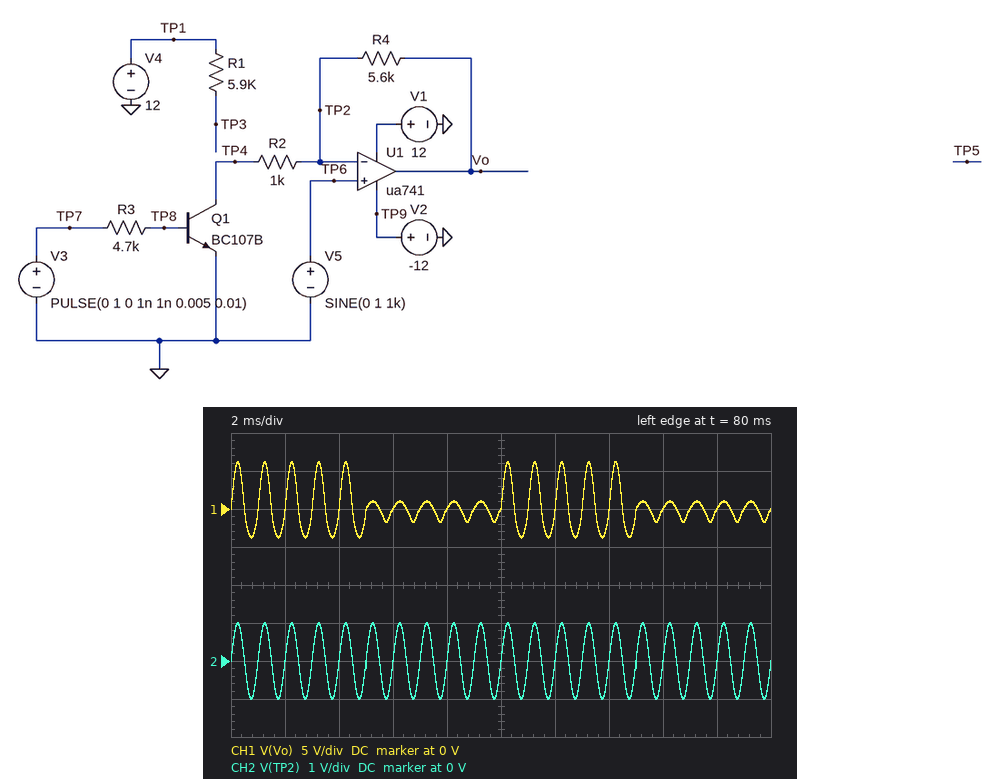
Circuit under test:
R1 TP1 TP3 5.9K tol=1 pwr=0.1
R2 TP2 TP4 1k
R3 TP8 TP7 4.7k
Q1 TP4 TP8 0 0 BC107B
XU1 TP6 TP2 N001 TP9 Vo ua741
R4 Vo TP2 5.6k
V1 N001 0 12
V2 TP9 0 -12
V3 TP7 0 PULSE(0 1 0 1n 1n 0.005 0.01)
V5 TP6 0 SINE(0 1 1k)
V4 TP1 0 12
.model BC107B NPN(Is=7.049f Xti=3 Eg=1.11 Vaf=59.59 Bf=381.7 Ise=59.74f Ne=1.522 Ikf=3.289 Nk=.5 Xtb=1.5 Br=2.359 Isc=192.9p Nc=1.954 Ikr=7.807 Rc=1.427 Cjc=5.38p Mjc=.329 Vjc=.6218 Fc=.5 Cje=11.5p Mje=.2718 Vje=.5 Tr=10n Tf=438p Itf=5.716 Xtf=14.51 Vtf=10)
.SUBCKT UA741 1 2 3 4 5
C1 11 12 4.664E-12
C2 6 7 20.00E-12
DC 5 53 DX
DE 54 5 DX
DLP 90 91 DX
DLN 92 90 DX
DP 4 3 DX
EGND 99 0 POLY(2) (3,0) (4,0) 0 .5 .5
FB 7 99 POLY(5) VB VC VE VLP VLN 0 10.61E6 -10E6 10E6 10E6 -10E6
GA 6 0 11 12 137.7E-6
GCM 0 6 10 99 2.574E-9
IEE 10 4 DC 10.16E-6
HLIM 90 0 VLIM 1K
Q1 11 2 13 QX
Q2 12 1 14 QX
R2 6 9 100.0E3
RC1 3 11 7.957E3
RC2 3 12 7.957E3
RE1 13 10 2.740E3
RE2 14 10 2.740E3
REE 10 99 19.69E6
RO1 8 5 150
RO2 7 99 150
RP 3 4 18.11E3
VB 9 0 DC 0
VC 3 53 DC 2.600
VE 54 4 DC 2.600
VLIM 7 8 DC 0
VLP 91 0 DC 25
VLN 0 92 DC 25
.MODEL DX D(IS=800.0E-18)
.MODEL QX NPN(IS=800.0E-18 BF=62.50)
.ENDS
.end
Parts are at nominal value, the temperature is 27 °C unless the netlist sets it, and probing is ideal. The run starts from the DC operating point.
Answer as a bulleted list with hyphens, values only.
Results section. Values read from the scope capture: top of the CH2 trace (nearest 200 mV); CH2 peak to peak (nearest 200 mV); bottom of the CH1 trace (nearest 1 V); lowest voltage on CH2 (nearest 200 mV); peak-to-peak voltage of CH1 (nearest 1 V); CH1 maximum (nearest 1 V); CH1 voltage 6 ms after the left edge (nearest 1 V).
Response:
- 1.0 V
- 2.0 V
- -4 V
- -1.0 V
- 10 V
- 6 V
- 0 V
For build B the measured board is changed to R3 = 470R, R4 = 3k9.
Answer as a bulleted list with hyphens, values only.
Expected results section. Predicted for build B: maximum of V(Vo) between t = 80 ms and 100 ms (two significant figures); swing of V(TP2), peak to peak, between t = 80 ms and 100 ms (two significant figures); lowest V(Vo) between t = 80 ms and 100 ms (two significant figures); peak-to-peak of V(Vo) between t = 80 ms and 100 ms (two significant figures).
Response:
- 4.8 V
- 2.0 V
- -4.9 V
- 9.7 V
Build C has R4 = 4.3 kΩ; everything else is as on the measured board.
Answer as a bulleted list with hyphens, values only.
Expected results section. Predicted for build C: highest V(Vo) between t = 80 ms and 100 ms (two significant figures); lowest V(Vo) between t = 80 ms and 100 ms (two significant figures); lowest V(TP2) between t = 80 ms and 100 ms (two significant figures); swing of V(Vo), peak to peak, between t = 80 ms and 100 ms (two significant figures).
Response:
- 5.0 V
- -3.1 V
- -1.0 V
- 8.1 V
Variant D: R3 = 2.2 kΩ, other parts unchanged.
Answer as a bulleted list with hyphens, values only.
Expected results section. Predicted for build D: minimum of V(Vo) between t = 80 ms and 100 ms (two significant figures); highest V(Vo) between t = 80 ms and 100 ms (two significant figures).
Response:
- -5.2 V
- 6.3 V
